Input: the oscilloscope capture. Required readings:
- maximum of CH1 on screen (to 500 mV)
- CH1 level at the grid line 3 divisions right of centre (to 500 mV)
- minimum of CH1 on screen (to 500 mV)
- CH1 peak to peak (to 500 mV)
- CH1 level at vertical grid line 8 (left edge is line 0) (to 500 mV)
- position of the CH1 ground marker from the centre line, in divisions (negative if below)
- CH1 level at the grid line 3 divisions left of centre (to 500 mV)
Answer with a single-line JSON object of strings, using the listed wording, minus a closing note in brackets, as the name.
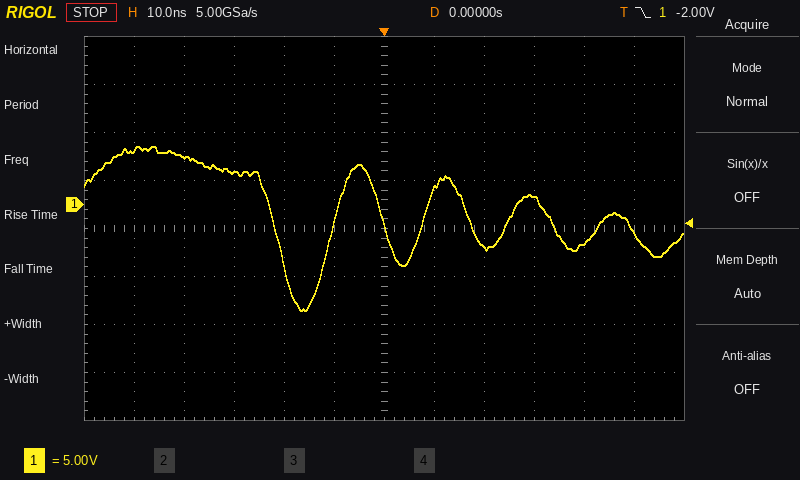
{"maximum of CH1 on screen": "6.0 V", "CH1 level at the grid line 3 divisions right of centre": "1.0 V", "minimum of CH1 on screen": "-11.0 V", "CH1 peak to peak": "17.0 V", "CH1 level at vertical grid line 8 (left edge is line 0)": "-4.5 V", "position of the CH1 ground marker from the centre line, in divisions": "+0.5 div", "CH1 level at the grid line 3 divisions left of centre": "3.5 V"}
